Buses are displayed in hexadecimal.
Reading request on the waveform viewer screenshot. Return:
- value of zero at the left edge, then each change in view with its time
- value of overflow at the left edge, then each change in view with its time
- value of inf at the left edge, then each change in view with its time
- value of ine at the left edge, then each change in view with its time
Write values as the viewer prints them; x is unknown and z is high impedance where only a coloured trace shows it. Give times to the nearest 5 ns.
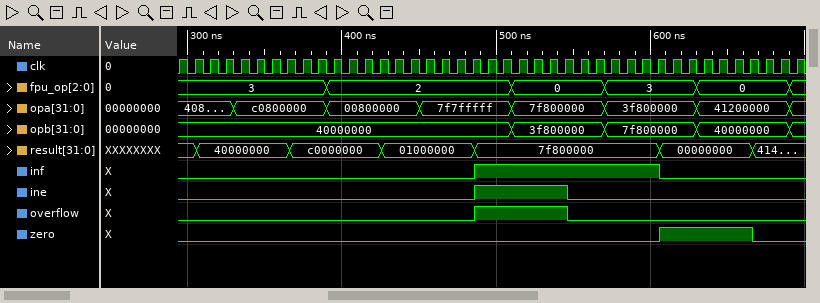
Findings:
0, 1 at 605 ns, 0 at 665 ns
0, 1 at 485 ns, 0 at 545 ns
0, 1 at 485 ns, 0 at 605 ns
0, 1 at 485 ns, 0 at 545 ns
